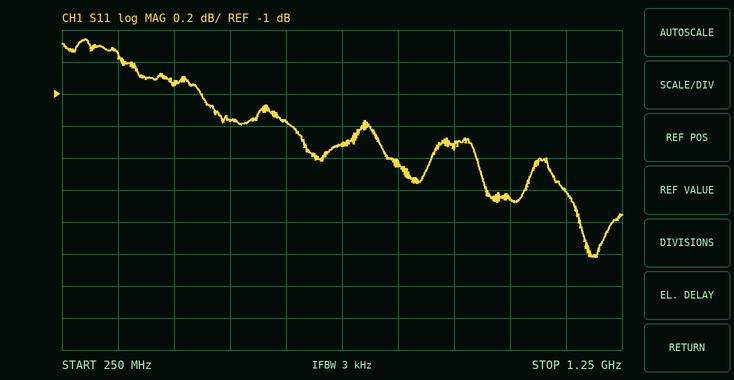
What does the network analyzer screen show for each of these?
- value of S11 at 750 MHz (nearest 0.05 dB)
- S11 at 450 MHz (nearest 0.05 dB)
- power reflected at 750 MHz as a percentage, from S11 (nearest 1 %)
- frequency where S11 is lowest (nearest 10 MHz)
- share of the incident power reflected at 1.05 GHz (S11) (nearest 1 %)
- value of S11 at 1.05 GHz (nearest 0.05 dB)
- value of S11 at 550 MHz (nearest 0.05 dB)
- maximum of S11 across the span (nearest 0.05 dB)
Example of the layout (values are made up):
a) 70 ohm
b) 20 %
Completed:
a) -1.30 dB
b) -0.95 dB
c) 74 %
d) 1.20 GHz
e) 68 %
f) -1.65 dB
g) -1.15 dB
h) -0.65 dB
